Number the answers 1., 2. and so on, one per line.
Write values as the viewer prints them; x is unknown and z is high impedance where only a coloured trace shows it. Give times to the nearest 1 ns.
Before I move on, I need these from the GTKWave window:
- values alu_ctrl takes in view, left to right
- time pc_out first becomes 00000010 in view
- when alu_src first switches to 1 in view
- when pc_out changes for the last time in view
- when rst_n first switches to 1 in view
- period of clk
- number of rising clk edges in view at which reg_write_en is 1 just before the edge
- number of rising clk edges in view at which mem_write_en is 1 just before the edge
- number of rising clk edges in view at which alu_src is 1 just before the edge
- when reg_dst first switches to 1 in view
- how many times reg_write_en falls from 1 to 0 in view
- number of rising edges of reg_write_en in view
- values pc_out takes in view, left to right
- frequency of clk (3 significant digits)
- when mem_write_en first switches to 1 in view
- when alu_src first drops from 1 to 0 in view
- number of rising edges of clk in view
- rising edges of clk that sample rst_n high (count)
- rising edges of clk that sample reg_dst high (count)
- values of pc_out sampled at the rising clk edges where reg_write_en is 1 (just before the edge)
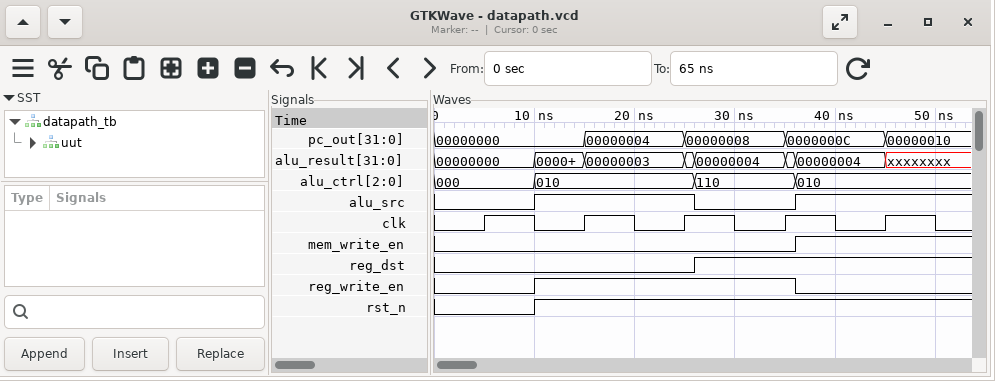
1. 000, 010, 110, 010
2. 45 ns
3. 10 ns
4. 45 ns
5. 10 ns
6. 10 ns
7. 3
8. 1
9. 3
10. 26 ns
11. 1
12. 1
13. 00000000, 00000004, 00000008, 0000000C, 00000010
14. 100 MHz
15. 36 ns
16. 26 ns
17. 5
18. 4
19. 2
20. 00000000, 00000004, 00000008
